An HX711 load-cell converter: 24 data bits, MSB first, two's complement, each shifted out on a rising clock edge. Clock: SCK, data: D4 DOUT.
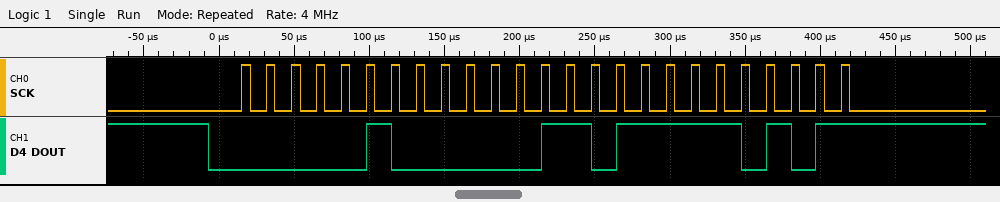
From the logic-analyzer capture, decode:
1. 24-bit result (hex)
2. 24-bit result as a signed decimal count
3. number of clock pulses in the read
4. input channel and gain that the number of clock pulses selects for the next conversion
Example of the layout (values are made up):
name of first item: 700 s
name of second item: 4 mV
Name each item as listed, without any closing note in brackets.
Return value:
24-bit result: 0x040DF5
24-bit result as a signed decimal count: 265717
number of clock pulses in the read: 25
input channel and gain that the number of clock pulses selects for the next conversion: channel A, gain 128
